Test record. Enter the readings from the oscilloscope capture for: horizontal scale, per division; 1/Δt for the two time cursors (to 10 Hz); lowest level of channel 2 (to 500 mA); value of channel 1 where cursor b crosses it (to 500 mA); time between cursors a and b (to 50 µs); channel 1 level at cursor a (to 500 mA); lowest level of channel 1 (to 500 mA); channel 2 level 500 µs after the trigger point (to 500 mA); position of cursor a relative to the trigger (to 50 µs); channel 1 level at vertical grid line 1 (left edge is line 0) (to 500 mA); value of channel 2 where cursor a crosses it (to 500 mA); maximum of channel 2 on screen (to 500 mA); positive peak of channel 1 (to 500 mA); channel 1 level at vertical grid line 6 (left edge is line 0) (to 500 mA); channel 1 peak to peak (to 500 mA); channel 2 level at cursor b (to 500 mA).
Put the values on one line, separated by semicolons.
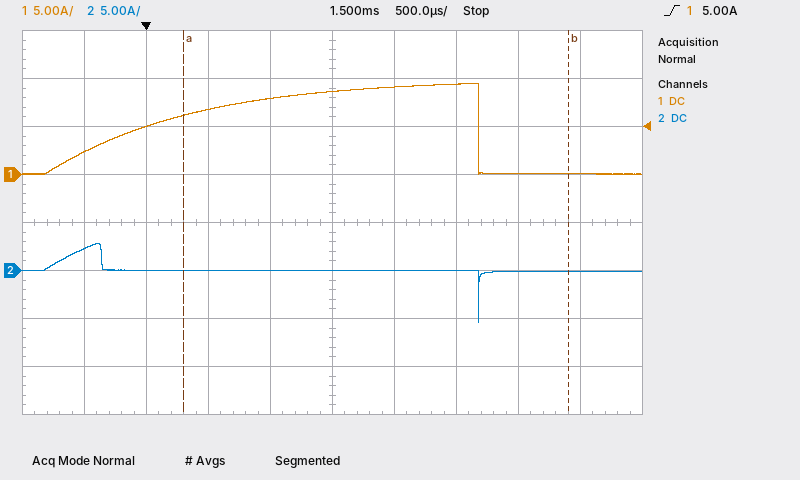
500 µs; 320 Hz; -5.5 A; 0.0 A; 3.10 ms; 6.0 A; 0.0 A; 0.0 A; +300 µs; 2.5 A; 0.0 A; 3.0 A; 9.5 A; 9.0 A; 9.5 A; 0.0 A
